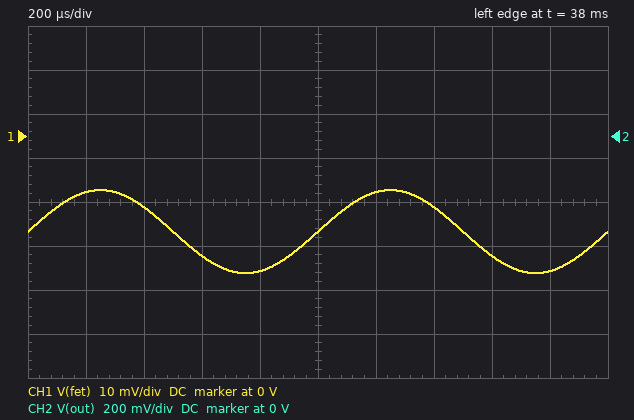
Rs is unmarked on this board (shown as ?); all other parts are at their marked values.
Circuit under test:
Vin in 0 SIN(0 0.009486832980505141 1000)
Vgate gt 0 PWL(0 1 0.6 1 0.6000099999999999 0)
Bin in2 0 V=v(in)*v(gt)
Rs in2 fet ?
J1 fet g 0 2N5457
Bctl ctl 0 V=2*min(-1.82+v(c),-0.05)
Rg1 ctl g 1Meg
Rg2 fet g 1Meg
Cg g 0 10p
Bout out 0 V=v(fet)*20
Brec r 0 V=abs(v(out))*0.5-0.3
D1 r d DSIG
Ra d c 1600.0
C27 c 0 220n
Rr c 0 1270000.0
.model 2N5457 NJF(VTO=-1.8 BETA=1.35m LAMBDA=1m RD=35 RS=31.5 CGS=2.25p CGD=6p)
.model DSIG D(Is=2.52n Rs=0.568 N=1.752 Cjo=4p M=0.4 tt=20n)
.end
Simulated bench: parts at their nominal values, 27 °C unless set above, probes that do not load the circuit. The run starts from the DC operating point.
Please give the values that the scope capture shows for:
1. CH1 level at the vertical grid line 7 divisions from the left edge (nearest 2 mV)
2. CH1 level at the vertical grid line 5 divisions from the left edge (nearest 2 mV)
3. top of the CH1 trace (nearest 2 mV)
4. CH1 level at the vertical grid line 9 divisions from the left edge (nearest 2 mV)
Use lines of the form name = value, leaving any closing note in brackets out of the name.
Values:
CH1 level at the vertical grid line 7 divisions from the left edge = -16 mV
CH1 level at the vertical grid line 5 divisions from the left edge = -22 mV
top of the CH1 trace = -12 mV
CH1 level at the vertical grid line 9 divisions from the left edge = -30 mV
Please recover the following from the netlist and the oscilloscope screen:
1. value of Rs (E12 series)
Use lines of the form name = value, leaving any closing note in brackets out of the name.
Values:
value of Rs = 12 kΩ
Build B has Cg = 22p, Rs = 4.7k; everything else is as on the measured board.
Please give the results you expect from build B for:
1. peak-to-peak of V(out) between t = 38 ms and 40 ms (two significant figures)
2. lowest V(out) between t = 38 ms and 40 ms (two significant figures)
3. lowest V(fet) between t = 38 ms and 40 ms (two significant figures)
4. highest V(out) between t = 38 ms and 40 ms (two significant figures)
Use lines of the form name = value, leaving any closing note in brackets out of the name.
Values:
peak-to-peak of V(out) between t = 38 ms and 40 ms = 380 mV
lowest V(out) between t = 38 ms and 40 ms = -360 mV
lowest V(fet) between t = 38 ms and 40 ms = -18 mV
highest V(out) between t = 38 ms and 40 ms = 18 mV
